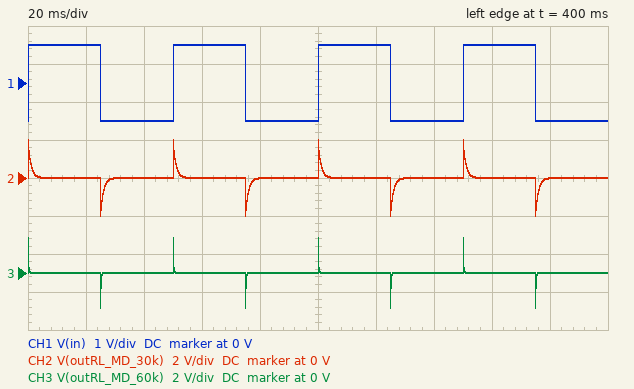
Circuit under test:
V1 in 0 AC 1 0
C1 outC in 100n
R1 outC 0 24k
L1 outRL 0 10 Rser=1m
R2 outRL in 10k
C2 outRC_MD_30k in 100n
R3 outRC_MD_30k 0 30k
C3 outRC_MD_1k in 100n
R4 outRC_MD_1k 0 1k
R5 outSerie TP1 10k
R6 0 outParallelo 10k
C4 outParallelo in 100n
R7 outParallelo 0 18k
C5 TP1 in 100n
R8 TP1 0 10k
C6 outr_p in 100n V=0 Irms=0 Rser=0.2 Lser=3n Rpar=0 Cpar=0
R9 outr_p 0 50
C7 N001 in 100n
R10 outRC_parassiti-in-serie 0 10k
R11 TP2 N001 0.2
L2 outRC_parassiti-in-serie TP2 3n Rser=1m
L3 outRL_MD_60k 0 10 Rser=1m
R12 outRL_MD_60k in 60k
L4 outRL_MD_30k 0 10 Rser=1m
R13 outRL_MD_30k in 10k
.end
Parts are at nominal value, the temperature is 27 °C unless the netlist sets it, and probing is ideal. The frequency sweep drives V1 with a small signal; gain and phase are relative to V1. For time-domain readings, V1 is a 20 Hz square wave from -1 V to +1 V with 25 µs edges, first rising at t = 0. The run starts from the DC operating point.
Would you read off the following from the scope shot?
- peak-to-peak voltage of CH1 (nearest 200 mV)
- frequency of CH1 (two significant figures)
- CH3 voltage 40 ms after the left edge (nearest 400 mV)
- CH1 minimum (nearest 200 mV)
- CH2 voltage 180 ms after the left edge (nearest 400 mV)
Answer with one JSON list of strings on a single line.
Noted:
["2.0 V", "20 Hz", "0 V", "-1.0 V", "0 V"]
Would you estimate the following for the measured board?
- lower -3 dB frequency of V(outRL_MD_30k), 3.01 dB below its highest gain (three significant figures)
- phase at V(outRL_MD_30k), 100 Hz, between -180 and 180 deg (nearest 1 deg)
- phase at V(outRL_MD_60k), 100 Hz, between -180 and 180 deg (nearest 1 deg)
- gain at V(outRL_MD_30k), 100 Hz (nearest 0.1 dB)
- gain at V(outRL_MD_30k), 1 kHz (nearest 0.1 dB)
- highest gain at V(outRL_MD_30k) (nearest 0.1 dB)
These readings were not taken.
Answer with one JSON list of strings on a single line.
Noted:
["159 Hz", "58 deg", "84 deg", "-5.5 dB", "-0.1 dB", "0 dB"]
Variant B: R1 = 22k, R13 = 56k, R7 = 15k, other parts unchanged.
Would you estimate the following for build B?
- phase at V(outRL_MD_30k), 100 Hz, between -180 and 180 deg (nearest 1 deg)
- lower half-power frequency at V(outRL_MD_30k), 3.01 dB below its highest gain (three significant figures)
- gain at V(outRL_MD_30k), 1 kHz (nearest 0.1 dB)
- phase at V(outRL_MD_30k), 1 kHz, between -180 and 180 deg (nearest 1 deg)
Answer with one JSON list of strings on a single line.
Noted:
["84 deg", "891 Hz", "-2.5 dB", "42 deg"]
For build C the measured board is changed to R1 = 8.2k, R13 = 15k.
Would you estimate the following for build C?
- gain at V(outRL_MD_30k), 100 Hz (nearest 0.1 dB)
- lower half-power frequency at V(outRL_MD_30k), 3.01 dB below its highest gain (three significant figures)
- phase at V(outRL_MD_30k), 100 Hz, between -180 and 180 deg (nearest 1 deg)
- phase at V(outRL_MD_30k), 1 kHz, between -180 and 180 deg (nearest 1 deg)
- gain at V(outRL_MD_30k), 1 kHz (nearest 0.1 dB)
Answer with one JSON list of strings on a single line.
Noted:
["-8.3 dB", "239 Hz", "67 deg", "13 deg", "-0.2 dB"]
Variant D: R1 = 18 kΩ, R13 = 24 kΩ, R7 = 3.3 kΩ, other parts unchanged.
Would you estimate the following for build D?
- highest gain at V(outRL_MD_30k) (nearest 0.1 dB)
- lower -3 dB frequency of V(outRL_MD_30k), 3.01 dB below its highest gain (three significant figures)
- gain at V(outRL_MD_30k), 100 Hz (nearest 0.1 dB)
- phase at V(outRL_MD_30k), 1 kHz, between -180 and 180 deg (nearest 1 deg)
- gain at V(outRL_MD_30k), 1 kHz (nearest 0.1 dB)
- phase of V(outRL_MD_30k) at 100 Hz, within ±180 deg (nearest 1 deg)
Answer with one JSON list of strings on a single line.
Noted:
["0 dB", "382 Hz", "-11.9 dB", "21 deg", "-0.6 dB", "75 deg"]
